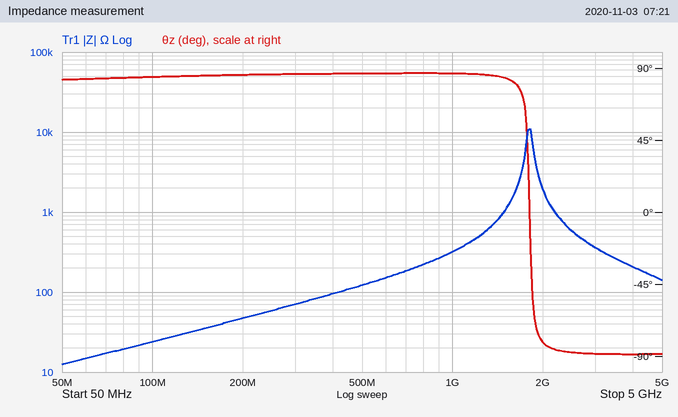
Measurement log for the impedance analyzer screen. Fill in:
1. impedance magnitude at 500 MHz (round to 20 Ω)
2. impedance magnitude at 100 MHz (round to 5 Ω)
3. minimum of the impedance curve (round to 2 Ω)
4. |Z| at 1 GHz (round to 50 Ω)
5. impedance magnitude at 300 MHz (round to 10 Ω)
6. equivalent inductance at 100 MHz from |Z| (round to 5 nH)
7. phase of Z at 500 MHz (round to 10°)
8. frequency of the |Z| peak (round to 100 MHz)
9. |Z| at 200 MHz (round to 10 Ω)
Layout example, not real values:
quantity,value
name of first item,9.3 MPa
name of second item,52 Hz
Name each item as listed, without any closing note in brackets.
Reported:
quantity,value
impedance magnitude at 500 MHz,120 Ω
impedance magnitude at 100 MHz,25 Ω
minimum of the impedance curve,12 Ω
|Z| at 1 GHz,300 Ω
impedance magnitude at 300 MHz,70 Ω
equivalent inductance at 100 MHz from |Z|,40 nH
phase of Z at 500 MHz,90°
frequency of the |Z| peak,1.8 GHz
|Z| at 200 MHz,50 Ω
